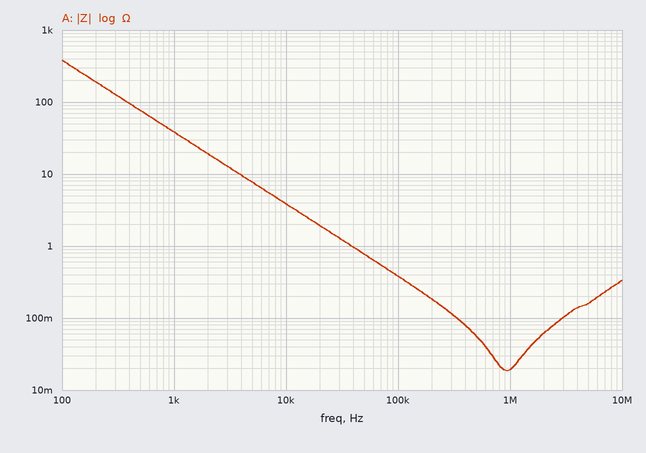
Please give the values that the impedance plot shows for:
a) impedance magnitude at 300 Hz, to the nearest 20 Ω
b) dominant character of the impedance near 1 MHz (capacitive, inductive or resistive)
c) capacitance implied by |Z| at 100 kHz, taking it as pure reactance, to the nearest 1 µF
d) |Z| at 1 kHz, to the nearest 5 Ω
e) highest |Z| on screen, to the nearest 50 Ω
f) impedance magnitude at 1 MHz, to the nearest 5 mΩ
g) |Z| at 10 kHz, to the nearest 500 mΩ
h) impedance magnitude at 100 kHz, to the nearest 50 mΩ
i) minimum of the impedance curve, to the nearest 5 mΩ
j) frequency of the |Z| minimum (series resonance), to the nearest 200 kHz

120 Ω
resistive
4 µF
40 Ω
400 Ω
20 mΩ
4.0 Ω
400 mΩ
20 mΩ
1.0 MHz
